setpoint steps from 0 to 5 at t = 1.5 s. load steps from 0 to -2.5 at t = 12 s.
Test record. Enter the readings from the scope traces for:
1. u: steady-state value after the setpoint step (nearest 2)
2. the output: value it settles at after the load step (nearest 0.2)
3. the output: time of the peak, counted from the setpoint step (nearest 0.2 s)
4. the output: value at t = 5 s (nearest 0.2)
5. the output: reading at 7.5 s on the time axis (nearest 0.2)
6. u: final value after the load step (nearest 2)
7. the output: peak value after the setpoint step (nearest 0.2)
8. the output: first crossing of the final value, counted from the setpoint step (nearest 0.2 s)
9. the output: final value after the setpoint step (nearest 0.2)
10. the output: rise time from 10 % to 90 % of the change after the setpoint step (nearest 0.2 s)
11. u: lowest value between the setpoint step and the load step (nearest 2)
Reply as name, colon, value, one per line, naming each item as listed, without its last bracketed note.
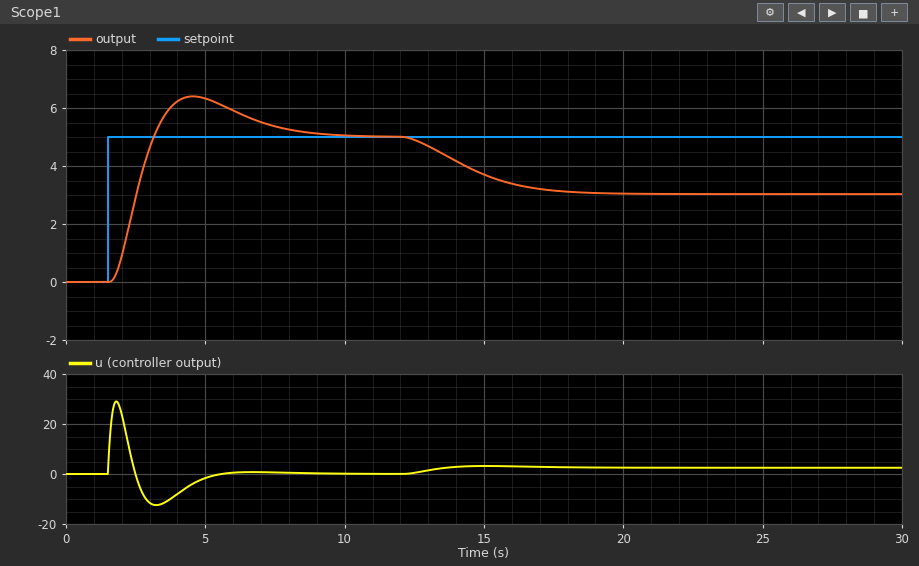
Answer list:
u: steady-state value after the setpoint step: 0
the output: value it settles at after the load step: 3.0
the output: time of the peak, counted from the setpoint step: 3.0 s
the output: value at t = 5 s: 6.4
the output: reading at 7.5 s on the time axis: 5.4
u: final value after the load step: 2
the output: peak value after the setpoint step: 6.4
the output: first crossing of the final value, counted from the setpoint step: 1.6 s
the output: final value after the setpoint step: 5.0
the output: rise time from 10 % to 90 % of the change after the setpoint step: 1.0 s
u: lowest value between the setpoint step and the load step: -12
